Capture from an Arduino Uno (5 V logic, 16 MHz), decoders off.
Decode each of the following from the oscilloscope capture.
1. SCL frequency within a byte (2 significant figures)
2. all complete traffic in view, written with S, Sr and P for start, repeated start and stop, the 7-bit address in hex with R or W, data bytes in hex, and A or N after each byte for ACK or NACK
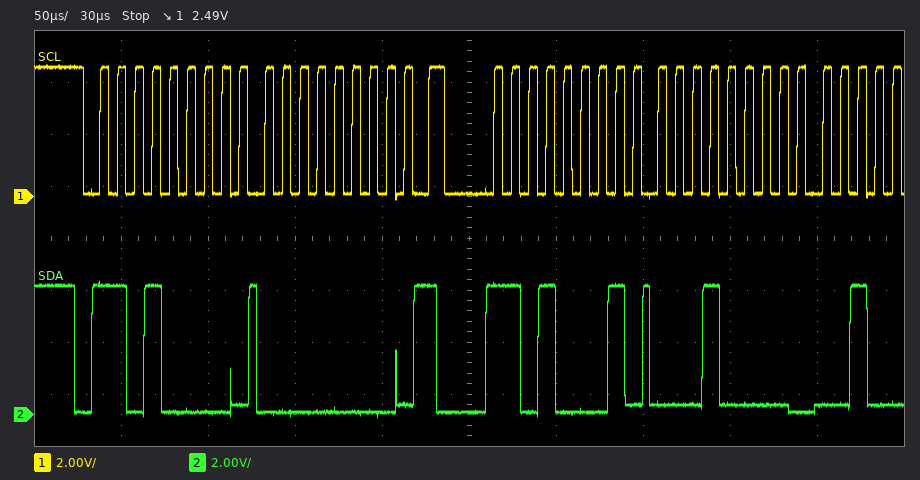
100 kHz
S 68W A 00 A Sr 68R A 10 A
